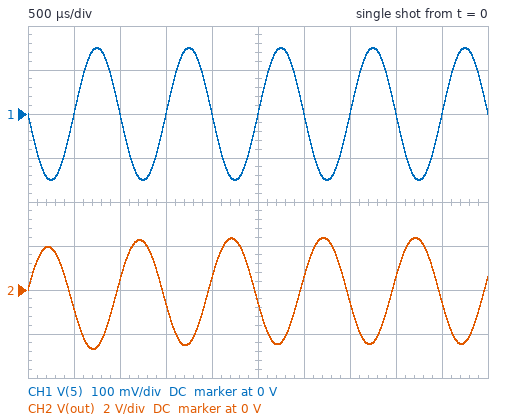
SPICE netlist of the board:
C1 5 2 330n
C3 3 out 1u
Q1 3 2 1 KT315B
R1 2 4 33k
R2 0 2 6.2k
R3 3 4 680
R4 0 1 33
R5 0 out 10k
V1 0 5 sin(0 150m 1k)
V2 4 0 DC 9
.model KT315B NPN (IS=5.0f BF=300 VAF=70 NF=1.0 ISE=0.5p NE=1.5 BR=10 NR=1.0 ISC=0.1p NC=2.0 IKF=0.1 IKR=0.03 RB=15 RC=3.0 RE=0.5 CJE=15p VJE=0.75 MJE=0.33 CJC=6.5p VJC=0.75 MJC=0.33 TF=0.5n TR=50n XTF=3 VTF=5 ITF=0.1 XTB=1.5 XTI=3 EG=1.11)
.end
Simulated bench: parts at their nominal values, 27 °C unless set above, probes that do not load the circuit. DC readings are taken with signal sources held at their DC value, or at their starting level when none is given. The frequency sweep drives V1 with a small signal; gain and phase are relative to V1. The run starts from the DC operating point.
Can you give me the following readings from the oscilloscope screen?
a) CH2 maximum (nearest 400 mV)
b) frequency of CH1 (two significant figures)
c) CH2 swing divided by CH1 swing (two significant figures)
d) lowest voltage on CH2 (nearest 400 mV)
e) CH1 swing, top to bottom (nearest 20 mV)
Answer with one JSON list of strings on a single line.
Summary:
["2.4 V", "1.0 kHz", "17", "-2.8 V", "300 mV"]
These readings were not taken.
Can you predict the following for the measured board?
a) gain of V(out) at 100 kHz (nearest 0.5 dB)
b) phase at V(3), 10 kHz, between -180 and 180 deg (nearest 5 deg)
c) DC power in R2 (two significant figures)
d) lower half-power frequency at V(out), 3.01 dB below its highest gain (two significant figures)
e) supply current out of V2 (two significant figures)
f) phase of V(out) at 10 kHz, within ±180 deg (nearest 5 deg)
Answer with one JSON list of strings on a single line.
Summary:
["24.5 dB", "0 deg", "150 µW", "230 Hz", "7.3 mA", "0 deg"]
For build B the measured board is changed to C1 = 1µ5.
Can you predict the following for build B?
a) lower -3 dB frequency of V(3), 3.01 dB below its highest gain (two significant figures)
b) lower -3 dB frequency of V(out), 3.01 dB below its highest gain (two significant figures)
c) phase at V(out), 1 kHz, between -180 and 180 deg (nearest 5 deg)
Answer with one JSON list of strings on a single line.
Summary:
["49 Hz", "54 Hz", "5 deg"]
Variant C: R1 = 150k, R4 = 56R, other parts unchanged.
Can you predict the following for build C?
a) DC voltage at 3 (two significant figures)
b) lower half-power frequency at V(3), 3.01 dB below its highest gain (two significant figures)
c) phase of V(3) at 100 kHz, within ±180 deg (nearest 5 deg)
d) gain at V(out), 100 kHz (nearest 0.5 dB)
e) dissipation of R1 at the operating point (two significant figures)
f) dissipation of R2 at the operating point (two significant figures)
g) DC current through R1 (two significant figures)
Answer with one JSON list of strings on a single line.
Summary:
["9.0 V", "62 MHz", "-85 deg", "-59.0 dB", "500 µW", "21 µW", "58 µA"]
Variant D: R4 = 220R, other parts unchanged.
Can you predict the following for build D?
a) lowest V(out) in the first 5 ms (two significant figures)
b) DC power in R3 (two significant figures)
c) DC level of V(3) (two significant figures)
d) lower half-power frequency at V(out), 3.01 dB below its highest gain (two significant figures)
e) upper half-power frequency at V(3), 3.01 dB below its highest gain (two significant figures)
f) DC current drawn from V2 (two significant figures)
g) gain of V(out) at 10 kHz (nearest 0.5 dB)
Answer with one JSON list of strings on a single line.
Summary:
["-440 mV", "3.9 mW", "7.4 V", "120 Hz", "92 MHz", "2.6 mA", "8.5 dB"]
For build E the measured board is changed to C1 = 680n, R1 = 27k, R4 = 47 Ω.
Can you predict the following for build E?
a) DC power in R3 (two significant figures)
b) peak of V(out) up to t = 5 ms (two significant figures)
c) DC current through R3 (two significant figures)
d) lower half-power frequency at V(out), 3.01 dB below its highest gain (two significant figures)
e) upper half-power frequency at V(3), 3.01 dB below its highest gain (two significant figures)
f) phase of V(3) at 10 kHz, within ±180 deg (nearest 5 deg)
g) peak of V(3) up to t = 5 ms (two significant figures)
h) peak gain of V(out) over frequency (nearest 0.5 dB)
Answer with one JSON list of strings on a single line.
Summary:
["51 mW", "1.8 V", "8.7 mA", "98 Hz", "42 MHz", "0 deg", "4.9 V", "22.0 dB"]
